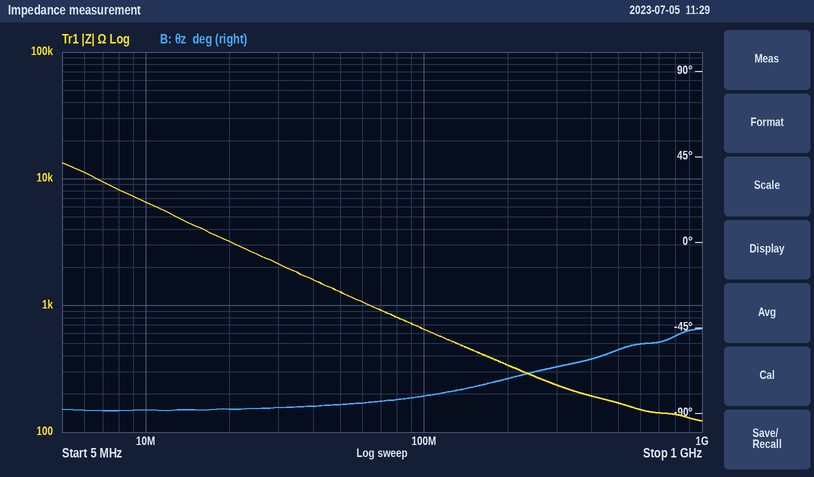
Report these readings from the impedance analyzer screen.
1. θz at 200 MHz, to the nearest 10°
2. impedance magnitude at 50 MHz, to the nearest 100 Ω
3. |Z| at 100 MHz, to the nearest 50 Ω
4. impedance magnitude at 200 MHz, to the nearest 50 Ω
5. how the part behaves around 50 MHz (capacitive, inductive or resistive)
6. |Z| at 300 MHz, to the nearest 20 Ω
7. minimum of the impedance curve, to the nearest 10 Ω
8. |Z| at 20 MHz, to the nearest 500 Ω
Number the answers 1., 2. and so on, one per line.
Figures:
1. -70°
2. 1.3 kΩ
3. 650 Ω
4. 350 Ω
5. capacitive
6. 240 Ω
7. 120 Ω
8. 3.0 kΩ
